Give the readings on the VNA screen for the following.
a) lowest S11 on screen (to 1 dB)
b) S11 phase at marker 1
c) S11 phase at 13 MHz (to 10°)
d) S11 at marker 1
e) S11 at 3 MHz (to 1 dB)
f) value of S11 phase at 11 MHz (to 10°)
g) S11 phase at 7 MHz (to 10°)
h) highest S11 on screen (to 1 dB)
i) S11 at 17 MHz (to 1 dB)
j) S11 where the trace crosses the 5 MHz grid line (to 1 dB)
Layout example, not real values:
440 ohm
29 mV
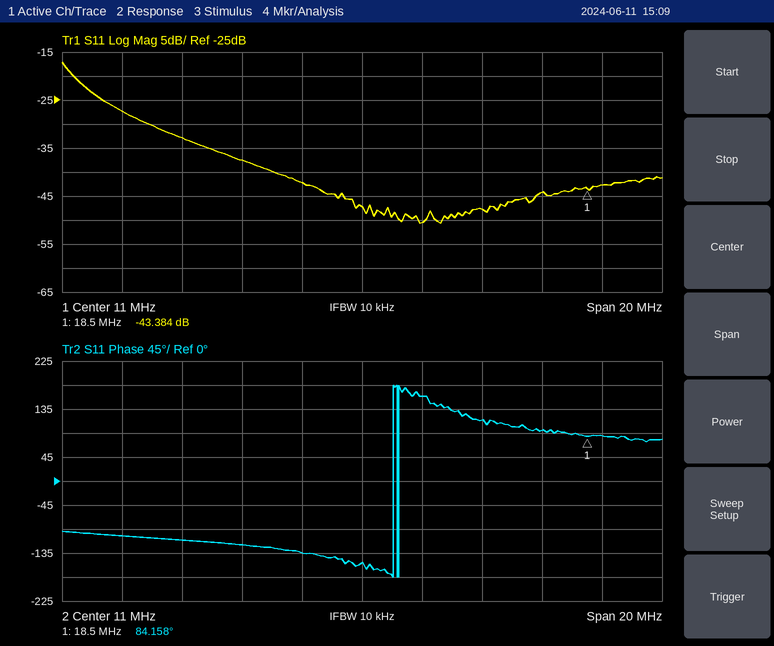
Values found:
-51 dB
84.158°
160°
-43.384 dB
-27 dB
-150°
-120°
-17 dB
-44 dB
-33 dB
